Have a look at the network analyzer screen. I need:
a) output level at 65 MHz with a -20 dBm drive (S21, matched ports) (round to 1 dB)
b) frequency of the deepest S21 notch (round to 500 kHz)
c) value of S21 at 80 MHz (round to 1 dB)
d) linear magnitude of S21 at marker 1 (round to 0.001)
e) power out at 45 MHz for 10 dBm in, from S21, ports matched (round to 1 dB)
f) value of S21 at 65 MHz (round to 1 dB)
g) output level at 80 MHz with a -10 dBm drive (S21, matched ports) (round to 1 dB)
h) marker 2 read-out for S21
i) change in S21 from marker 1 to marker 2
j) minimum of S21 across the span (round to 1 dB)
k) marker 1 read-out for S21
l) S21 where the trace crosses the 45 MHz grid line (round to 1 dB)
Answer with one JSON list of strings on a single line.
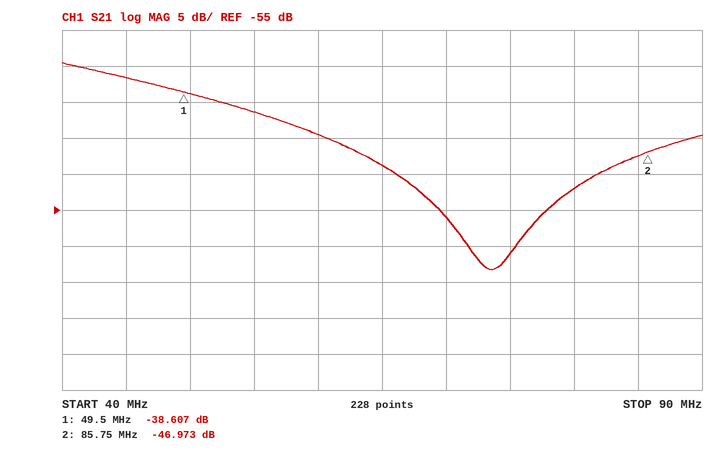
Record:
["-69 dBm", "73.5 MHz", "-52 dB", "0.012", "-27 dBm", "-49 dB", "-62 dBm", "-46.973 dB", "-8.366 dB", "-63 dB", "-38.607 dB", "-37 dB"]
